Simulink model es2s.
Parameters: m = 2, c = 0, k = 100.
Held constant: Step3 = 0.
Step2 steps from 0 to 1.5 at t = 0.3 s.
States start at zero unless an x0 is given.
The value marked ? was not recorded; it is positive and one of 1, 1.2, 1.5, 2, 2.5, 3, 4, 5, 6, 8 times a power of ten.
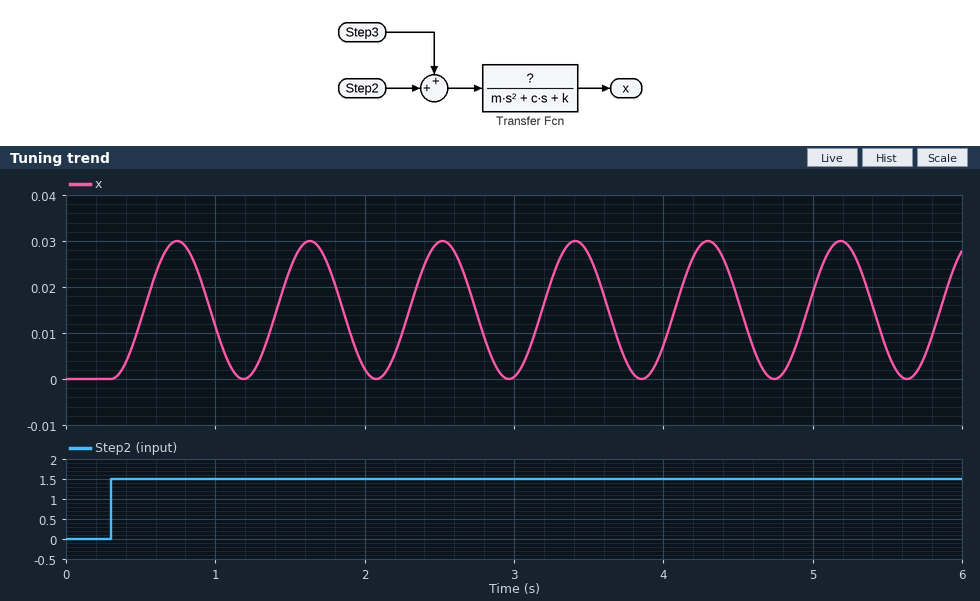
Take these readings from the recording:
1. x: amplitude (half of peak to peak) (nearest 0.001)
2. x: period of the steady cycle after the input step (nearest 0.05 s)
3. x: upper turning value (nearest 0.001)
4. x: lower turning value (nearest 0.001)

0.015
0.90 s
0.030
0.000
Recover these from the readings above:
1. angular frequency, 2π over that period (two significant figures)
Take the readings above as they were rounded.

7.0 rad/s
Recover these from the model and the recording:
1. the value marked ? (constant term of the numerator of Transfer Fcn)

1
